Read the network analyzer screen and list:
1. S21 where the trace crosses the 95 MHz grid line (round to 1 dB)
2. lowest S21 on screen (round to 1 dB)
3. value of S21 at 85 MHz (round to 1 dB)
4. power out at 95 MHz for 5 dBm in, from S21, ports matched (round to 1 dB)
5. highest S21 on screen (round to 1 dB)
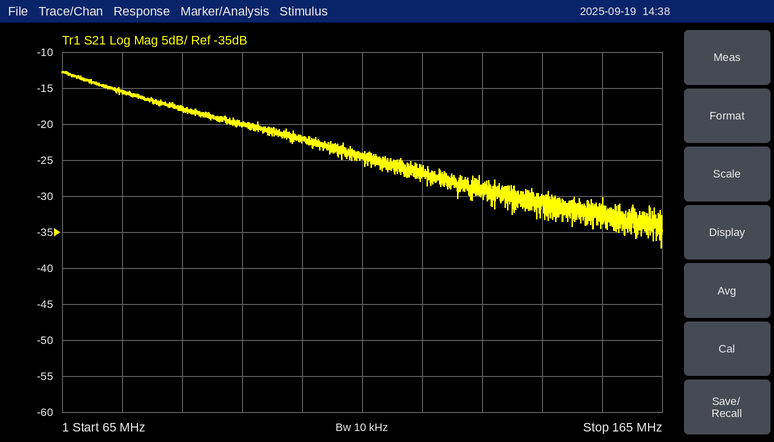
-20 dB
-37 dB
-18 dB
-15 dBm
-13 dB
